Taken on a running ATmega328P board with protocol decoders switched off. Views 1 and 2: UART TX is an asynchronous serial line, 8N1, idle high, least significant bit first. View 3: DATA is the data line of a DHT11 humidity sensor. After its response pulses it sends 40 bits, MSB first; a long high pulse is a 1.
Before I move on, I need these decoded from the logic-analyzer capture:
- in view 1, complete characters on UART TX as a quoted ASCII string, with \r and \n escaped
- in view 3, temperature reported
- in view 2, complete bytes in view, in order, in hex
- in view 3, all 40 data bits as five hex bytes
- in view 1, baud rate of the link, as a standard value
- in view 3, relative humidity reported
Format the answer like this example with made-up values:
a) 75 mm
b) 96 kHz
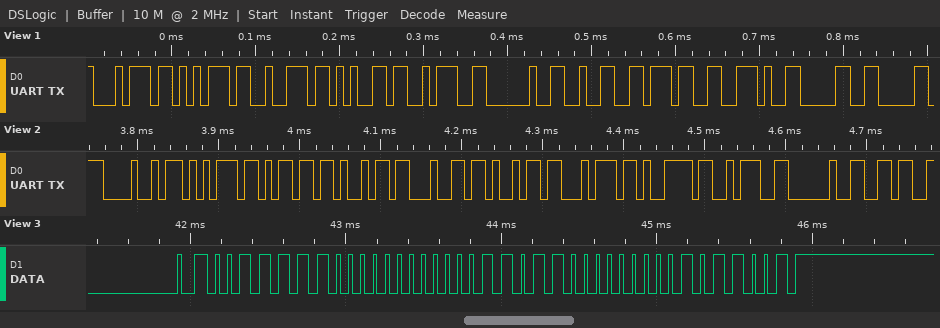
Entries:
a) "ture: 27.0"
b) 27.0 °C
c) 0x48 0x75 0x6D 0x69 0x64 0x69 0x74 0x79 0x3A 0x20 0x36
d) 3E 00 1B 00 59
e) 115200 baud
f) 62 %
